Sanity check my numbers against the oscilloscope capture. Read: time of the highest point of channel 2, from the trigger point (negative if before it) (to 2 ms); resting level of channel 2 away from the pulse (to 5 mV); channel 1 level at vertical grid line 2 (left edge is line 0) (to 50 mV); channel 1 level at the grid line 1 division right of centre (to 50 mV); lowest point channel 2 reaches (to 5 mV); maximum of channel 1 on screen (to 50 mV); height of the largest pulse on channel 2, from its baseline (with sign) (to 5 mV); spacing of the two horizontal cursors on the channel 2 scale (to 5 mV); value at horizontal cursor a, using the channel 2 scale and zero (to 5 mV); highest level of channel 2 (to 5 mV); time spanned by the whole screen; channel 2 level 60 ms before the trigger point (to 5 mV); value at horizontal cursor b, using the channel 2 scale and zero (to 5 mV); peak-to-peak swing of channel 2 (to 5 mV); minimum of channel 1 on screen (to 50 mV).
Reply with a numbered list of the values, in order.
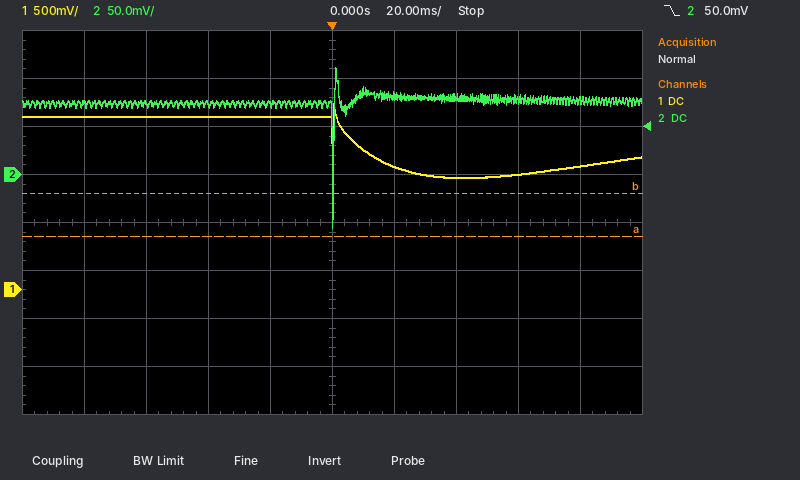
1. +2 ms
2. 75 mV
3. 1.80 V
4. 1.30 V
5. -55 mV
6. 1.95 V
7. -130 mV
8. 45 mV
9. -65 mV
10. 110 mV
11. 200 ms
12. 75 mV
13. -20 mV
14. 165 mV
15. 1.15 V
